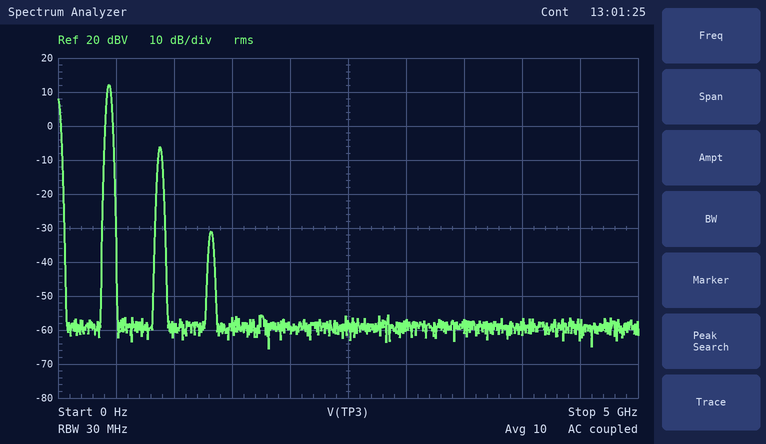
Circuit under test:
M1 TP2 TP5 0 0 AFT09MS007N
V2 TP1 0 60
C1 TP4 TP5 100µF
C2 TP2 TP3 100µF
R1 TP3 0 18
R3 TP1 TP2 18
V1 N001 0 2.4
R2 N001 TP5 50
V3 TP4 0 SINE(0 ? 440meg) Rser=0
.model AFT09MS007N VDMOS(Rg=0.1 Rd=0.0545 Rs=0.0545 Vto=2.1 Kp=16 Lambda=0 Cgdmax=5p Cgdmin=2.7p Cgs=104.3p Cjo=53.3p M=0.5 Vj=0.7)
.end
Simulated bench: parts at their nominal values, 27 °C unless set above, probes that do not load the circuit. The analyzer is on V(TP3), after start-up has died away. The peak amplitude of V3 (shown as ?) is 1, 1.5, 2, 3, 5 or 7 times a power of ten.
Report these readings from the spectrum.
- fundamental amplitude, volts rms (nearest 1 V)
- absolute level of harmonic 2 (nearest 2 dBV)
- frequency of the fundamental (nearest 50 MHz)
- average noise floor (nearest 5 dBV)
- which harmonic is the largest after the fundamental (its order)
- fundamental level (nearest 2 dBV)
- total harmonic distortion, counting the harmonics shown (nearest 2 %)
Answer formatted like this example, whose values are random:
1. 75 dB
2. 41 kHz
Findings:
1. 4 V
2. -6 dBV
3. 450 MHz
4. -60 dBV
5. 2
6. 12 dBV
7. 12 %
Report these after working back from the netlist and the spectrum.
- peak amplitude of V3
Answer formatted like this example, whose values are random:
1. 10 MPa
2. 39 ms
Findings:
1. 200 mV
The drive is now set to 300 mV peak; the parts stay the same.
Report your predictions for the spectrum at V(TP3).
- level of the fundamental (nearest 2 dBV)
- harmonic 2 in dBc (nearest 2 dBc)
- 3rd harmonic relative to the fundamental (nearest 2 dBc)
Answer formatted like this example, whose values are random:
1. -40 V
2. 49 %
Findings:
1. 16 dBV
2. -14 dBc
3. -38 dBc
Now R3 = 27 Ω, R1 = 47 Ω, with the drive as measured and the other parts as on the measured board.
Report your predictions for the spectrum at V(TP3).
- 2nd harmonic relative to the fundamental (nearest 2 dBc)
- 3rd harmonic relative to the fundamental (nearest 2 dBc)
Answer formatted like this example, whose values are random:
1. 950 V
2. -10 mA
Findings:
1. -20 dBc
2. -42 dBc
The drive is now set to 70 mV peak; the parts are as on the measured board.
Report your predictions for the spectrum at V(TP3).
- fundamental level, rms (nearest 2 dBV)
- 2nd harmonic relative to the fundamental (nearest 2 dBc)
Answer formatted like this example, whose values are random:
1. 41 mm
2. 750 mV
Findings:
1. 4 dBV
2. -28 dBc
